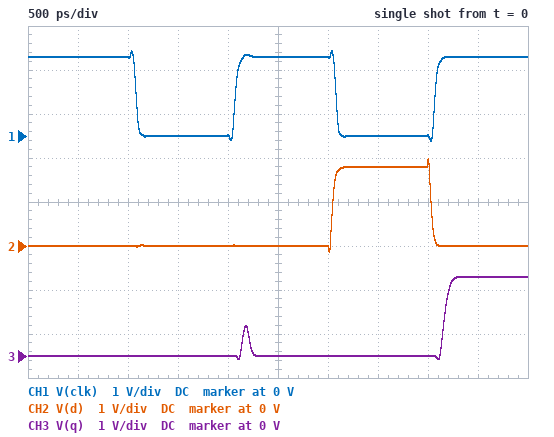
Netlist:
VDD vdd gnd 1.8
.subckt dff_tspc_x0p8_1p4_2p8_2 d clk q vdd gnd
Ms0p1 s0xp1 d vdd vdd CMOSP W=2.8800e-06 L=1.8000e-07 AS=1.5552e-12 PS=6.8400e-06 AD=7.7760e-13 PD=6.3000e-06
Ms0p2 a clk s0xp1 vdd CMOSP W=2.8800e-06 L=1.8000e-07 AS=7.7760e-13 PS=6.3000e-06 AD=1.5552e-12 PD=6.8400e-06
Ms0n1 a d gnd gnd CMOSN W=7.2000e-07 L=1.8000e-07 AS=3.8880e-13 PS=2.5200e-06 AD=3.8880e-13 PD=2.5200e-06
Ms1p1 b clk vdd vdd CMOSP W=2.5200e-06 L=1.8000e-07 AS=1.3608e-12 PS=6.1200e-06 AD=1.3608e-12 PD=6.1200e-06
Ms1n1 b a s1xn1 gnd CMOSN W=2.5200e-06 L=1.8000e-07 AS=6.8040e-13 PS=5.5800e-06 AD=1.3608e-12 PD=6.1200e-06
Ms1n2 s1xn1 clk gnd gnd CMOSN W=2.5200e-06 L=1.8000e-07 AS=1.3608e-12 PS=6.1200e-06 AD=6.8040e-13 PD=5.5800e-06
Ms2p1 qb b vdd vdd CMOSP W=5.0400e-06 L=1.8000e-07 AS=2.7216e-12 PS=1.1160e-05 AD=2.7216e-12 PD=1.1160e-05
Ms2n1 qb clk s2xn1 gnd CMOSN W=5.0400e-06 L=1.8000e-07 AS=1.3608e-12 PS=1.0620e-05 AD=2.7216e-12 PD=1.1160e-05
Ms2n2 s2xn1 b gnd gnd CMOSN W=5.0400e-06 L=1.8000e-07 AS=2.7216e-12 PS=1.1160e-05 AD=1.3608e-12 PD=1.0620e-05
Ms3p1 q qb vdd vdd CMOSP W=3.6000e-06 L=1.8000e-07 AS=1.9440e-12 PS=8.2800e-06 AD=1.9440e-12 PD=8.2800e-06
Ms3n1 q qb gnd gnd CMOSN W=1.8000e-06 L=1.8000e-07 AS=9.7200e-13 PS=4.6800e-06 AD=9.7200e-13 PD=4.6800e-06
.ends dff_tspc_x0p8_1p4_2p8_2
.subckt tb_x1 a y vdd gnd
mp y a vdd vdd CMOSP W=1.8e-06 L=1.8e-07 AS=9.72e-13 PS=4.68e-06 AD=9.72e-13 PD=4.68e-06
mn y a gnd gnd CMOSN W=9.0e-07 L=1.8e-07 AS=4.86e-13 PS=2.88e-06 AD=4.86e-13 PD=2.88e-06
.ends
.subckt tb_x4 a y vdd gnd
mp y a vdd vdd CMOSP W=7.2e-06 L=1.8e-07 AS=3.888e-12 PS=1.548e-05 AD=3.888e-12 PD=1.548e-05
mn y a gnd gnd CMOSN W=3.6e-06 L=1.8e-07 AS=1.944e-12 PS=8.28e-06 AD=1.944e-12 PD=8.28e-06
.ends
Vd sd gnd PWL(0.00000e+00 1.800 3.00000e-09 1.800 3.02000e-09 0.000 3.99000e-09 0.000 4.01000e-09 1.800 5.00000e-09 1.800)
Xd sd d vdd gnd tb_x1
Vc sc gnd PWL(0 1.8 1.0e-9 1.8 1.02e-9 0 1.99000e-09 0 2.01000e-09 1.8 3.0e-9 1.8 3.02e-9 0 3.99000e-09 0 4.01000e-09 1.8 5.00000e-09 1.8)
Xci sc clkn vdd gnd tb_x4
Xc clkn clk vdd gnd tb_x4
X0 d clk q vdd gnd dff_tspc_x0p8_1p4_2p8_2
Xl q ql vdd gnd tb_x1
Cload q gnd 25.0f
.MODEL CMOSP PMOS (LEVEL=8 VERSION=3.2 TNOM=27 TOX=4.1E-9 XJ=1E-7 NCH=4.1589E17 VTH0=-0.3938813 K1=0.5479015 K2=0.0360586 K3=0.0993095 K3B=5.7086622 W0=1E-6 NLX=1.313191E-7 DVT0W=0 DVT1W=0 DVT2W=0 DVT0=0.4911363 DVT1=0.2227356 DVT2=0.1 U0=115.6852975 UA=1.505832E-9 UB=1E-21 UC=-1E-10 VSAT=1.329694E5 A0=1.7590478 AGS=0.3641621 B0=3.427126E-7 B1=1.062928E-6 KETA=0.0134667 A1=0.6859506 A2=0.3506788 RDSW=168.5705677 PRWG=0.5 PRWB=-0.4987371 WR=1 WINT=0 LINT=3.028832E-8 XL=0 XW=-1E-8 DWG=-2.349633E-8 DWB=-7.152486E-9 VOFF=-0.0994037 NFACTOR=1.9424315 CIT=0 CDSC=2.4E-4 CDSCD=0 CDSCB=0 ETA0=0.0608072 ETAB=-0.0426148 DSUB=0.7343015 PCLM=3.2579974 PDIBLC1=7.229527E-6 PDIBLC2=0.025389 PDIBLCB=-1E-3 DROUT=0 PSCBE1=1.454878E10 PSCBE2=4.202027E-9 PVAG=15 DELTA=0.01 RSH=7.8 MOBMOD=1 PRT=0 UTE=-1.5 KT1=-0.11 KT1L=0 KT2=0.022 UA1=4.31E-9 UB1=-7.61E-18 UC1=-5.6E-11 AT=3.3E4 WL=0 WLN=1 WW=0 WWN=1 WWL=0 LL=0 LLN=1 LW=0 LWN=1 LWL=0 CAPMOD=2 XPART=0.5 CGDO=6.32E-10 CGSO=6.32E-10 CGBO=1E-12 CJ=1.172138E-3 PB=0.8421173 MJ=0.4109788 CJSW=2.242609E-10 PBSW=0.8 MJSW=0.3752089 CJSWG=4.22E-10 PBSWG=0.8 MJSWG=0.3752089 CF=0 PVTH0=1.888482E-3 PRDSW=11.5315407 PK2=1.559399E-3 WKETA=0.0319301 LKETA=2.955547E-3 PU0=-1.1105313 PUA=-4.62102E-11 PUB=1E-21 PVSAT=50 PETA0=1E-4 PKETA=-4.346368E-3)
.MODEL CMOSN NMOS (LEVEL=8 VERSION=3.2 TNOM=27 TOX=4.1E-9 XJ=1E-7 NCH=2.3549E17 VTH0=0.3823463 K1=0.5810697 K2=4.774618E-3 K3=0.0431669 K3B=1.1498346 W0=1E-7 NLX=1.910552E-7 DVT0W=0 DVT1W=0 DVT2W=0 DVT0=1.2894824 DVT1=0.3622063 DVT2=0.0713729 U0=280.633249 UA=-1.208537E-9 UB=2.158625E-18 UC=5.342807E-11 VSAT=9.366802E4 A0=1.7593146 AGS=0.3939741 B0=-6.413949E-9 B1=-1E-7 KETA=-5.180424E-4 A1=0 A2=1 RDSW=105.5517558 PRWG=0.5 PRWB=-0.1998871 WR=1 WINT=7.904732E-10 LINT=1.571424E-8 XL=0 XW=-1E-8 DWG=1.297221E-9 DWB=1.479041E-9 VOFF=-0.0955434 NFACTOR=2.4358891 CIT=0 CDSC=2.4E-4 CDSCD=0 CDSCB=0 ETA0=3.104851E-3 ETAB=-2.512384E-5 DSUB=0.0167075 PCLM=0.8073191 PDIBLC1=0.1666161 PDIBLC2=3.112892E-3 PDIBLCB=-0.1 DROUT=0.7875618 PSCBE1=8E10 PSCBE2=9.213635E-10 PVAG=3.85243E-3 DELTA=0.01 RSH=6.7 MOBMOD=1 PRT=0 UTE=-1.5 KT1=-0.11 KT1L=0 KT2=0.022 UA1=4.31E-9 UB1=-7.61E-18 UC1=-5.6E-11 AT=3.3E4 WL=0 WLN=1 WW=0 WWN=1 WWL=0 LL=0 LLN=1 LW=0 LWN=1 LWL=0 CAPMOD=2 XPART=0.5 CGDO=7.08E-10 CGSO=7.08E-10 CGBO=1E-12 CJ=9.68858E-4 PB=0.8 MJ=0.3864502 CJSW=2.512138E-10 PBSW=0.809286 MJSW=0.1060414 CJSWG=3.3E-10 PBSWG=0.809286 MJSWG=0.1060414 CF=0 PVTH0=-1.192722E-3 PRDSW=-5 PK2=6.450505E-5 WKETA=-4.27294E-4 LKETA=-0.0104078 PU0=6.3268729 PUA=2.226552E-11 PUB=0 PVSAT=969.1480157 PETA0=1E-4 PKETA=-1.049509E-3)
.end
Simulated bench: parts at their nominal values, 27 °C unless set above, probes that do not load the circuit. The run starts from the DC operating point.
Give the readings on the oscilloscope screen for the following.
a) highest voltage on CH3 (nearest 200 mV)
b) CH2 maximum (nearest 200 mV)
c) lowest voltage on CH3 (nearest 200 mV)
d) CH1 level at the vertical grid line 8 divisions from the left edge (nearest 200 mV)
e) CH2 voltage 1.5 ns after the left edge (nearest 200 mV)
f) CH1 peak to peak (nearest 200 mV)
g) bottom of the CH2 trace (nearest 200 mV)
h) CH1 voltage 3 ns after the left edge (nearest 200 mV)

1.8 V
2.0 V
0 V
0 V
0 V
2.0 V
-200 mV
1.8 V
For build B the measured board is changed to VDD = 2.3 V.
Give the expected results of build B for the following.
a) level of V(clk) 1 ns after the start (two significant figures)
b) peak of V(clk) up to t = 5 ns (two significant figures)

2.3 V
2.4 V
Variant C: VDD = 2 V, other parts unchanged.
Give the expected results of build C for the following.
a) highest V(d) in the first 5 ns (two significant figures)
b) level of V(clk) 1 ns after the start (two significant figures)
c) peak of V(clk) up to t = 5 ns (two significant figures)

2.2 V
2.0 V
2.1 V
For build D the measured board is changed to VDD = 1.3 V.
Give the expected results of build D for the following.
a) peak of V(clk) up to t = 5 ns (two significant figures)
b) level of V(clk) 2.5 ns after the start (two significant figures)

1.4 V
1.3 V
